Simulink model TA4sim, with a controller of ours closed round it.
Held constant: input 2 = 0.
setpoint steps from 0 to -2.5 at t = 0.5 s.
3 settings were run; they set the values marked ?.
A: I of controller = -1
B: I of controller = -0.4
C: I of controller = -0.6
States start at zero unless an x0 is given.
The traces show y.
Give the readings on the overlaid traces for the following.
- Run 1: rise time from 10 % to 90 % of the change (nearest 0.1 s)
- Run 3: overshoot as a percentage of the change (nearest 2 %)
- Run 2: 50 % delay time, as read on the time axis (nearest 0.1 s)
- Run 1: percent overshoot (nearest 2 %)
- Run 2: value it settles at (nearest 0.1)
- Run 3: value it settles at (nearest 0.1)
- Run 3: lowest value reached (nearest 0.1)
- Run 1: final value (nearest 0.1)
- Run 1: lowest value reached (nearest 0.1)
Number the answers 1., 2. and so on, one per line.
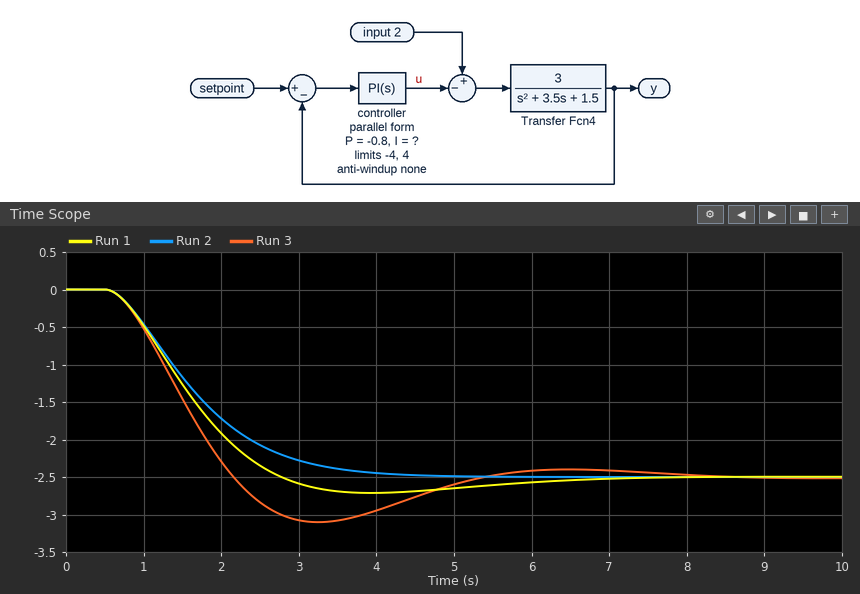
1. 1.5 s
2. 24 %
3. 1.6 s
4. 8 %
5. -2.5
6. -2.5
7. -3.1
8. -2.5
9. -2.7
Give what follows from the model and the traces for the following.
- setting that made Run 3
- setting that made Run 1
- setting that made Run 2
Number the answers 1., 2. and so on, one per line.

1. A
2. C
3. B
